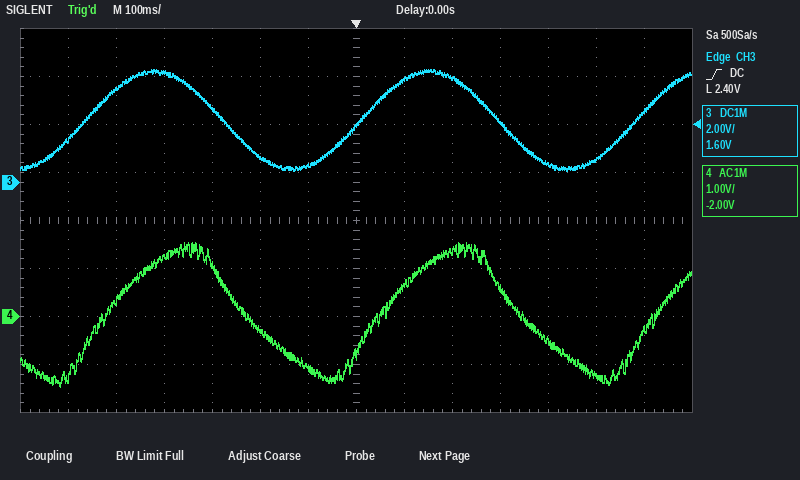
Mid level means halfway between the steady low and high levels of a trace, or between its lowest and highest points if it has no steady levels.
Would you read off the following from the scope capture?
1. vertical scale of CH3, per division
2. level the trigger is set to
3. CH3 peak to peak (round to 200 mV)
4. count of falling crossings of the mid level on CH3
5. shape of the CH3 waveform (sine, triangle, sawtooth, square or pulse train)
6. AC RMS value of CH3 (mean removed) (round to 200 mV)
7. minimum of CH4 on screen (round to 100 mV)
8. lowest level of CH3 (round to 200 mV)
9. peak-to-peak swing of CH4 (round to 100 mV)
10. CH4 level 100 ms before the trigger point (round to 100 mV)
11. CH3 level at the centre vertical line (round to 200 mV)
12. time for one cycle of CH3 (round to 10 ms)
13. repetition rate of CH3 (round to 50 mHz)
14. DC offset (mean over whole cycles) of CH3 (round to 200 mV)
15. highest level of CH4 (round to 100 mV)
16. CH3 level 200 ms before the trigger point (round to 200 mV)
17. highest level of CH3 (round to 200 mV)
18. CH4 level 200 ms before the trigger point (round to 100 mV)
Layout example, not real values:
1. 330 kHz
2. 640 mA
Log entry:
1. 2 V
2. 2.40 V
3. 4.2 V
4. 2
5. sine
6. 1.4 V
7. -1.5 V
8. 400 mV
9. 3.0 V
10. -1.1 V
11. 2.4 V
12. 570 ms
13. 1.75 Hz
14. 2.6 V
15. 1.5 V
16. 1.0 V
17. 4.6 V
18. -300 mV
